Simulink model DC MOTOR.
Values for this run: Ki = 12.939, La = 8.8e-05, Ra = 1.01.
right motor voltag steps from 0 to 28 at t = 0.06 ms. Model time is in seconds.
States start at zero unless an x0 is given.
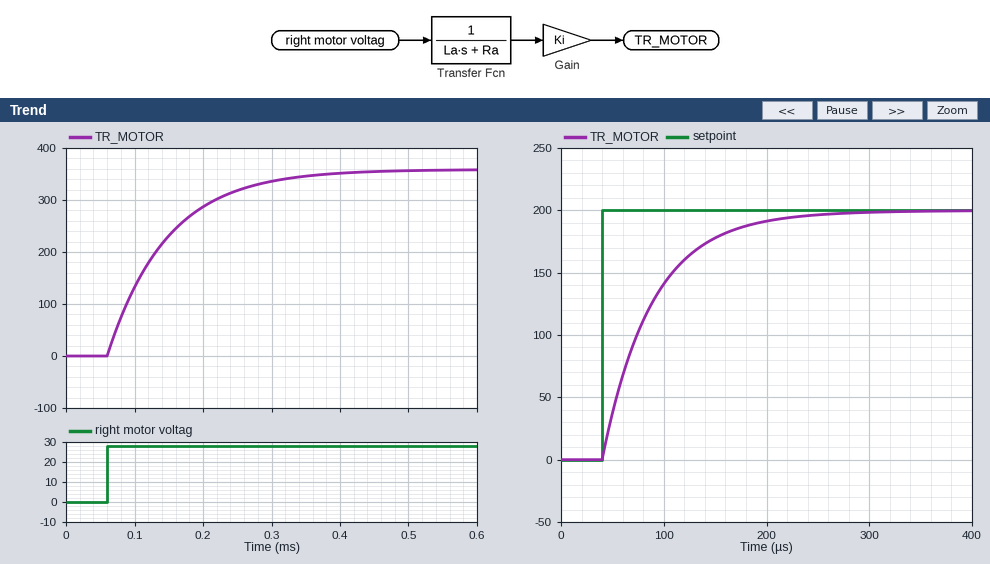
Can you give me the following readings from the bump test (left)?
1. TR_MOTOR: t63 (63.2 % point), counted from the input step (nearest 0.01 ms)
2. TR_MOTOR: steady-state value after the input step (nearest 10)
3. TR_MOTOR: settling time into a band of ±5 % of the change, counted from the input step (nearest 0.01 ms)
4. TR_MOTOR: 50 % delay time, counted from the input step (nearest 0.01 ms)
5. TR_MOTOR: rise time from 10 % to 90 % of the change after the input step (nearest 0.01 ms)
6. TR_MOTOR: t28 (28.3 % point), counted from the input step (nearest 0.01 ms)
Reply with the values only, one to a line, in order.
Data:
0.09 ms
360
0.26 ms
0.06 ms
0.19 ms
0.03 ms
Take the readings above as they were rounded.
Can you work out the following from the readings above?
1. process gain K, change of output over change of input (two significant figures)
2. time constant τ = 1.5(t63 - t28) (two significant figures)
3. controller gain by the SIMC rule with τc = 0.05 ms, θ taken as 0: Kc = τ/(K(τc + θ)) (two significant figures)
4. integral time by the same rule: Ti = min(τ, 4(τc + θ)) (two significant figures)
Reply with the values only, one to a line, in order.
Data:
13
0.090 ms
0.14
0.090 ms
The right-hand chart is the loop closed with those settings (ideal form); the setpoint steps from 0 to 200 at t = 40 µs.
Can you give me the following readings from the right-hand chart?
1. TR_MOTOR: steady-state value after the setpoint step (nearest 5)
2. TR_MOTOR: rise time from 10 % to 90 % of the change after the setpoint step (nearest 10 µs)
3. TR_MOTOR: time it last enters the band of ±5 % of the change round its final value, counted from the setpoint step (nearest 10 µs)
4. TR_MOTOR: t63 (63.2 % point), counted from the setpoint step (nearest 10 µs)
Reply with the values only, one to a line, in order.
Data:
200
110 µs
150 µs
50 µs
